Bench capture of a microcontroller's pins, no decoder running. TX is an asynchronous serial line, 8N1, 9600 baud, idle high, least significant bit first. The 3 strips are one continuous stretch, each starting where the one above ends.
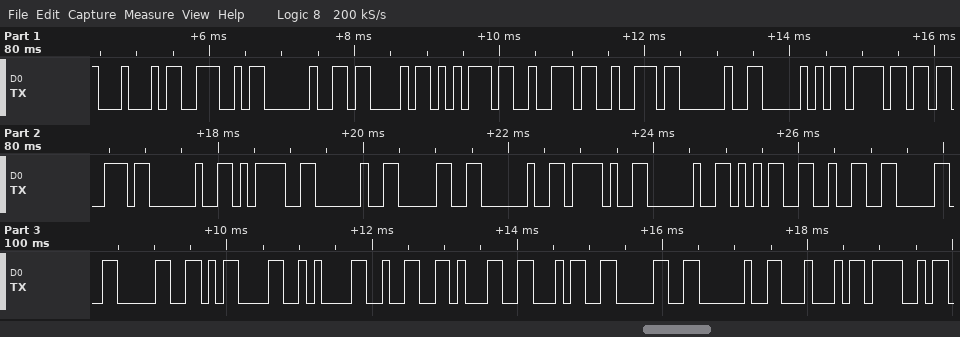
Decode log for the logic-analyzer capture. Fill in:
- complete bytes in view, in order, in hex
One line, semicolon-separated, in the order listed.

0x44 0x4E 0x20 0x43 0x75 0x72 0x72 0x20 0x50 0x6F 0x73 0x20 0x3D 0x20 0x30 0x20 0x2F 0x20 0x35 0x32 0x30 0x30 0x0D 0x0A 0x32 0x31 0x34 0x30 0x20 0x44 0x4F
